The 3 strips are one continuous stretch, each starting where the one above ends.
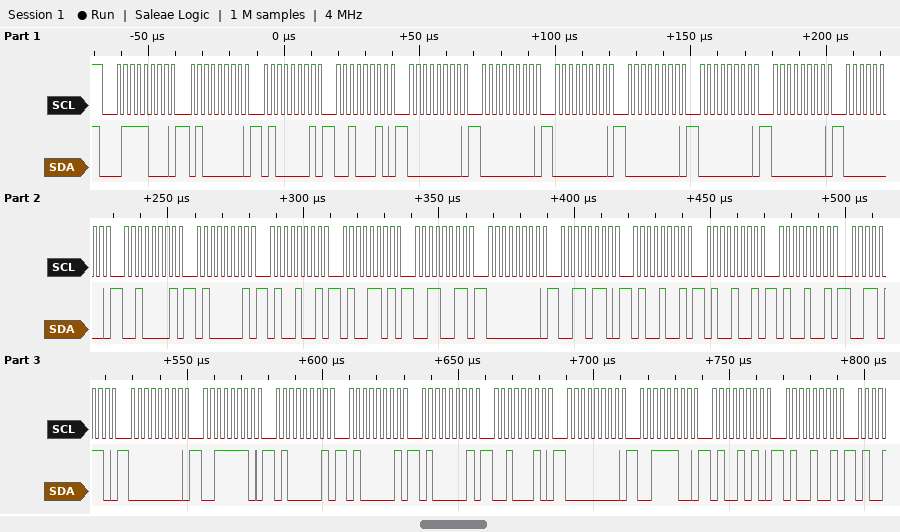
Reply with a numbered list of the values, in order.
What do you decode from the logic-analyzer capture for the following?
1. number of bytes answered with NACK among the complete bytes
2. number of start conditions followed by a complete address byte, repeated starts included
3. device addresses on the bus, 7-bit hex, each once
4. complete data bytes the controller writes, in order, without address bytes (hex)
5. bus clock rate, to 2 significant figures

1. 0
2. 1
3. 0x3C
4. 40 41 22 00 00 00 00 00 00 00 21 41 49 4D 33 00 36 49 49 49 36 00 3E 41 41 41 22 00 3C 4A 49
5. 400 kHz
